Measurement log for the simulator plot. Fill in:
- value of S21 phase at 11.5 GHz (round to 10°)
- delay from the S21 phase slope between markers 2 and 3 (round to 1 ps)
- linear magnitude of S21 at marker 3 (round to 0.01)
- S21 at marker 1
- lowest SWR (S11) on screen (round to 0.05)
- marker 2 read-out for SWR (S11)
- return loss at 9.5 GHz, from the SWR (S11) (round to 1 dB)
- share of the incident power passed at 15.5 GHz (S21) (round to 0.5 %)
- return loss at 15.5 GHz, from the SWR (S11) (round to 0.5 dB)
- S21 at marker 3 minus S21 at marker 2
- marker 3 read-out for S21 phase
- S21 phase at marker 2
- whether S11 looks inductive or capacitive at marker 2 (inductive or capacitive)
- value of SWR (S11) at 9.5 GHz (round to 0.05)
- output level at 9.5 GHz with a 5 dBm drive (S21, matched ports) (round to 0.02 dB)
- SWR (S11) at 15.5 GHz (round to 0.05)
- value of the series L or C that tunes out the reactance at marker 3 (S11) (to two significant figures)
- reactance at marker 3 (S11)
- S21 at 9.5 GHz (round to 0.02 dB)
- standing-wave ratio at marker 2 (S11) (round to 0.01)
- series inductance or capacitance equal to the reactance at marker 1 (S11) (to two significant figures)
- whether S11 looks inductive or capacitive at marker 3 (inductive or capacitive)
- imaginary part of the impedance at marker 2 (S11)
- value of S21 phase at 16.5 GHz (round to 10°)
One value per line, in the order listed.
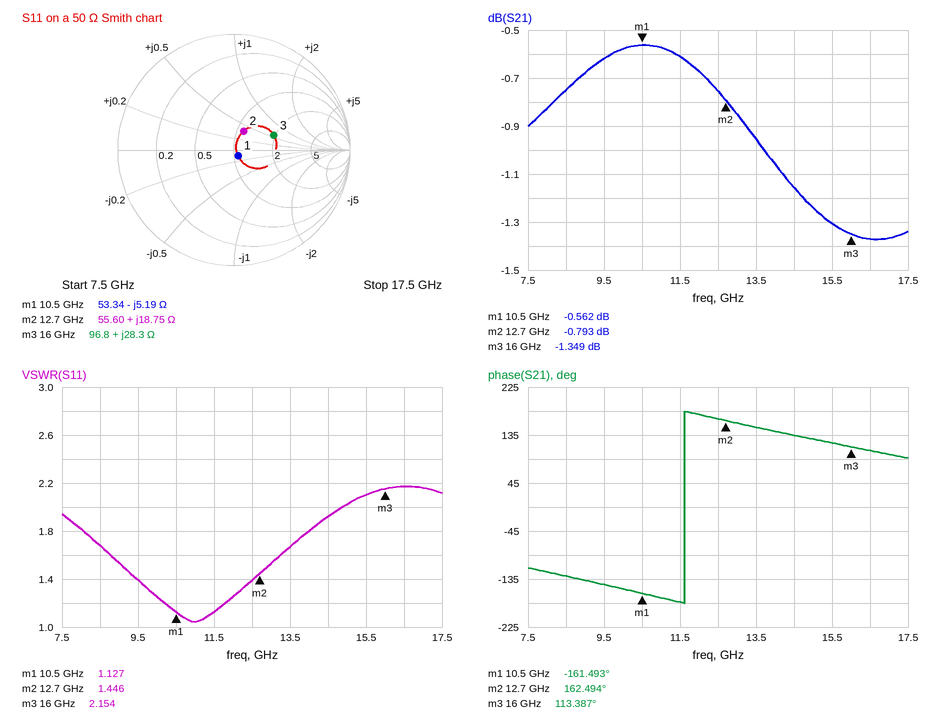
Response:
-180°
41 ps
0.86
-0.562 dB
1.05
1.446
16 dB
74.0 %
9.0 dB
-0.556 dB
113.387°
162.494°
inductive
1.40
4.38 dBm
2.10
350 fF
+28.3 Ω
-0.62 dB
1.45
2.9 pF
inductive
+18.75 Ω
110°
